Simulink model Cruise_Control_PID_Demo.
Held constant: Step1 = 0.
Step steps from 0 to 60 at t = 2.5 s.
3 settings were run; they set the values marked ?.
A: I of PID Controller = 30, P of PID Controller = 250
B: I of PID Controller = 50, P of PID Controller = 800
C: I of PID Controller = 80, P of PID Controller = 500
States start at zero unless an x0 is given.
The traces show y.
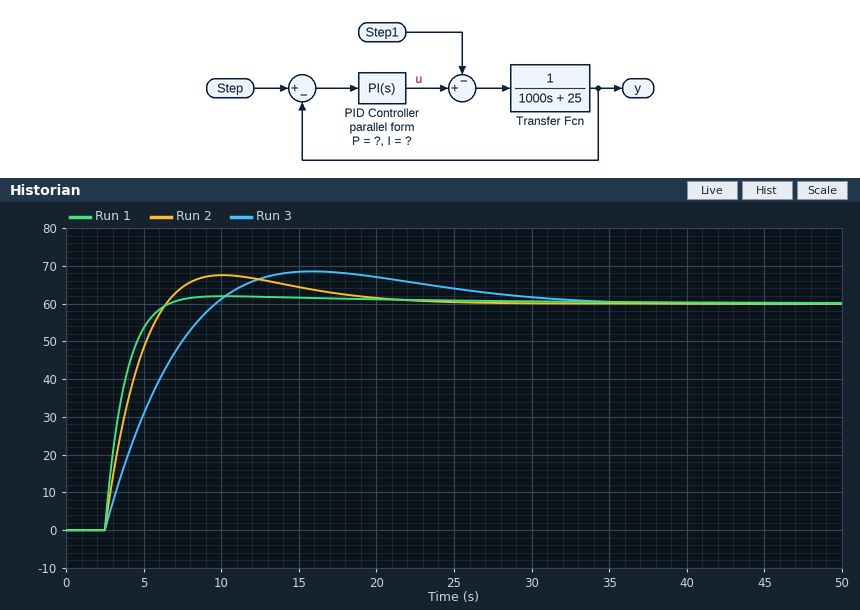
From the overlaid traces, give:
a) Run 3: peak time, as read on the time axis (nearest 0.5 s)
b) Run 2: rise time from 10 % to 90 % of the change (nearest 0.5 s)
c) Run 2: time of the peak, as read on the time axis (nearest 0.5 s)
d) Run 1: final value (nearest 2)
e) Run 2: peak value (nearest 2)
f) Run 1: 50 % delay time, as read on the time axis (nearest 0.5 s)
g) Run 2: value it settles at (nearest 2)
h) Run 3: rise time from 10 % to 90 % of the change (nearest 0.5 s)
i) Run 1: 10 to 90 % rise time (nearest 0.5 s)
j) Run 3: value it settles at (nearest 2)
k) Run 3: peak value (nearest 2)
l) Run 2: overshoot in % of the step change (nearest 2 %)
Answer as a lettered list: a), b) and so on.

a) 16.0 s
b) 3.0 s
c) 10.0 s
d) 60
e) 68
f) 3.5 s
g) 60
h) 5.5 s
i) 2.5 s
j) 60
k) 68
l) 12 %
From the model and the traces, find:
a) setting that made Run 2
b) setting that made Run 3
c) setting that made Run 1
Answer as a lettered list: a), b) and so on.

a) C
b) A
c) B
